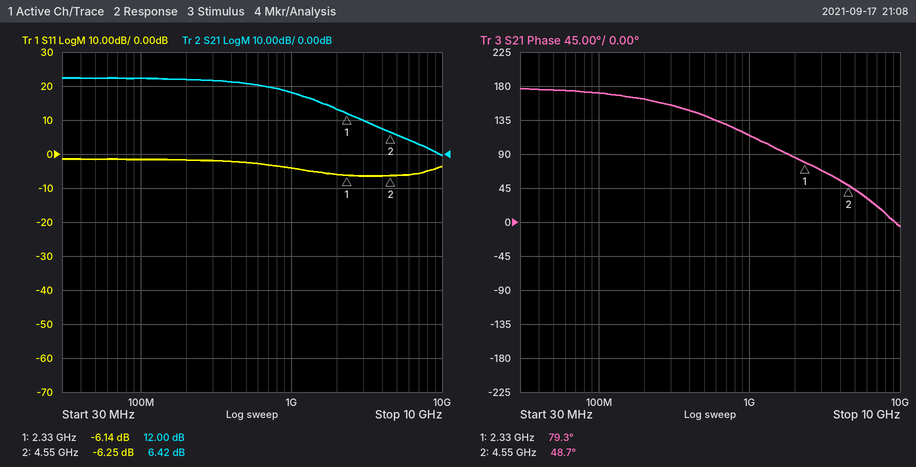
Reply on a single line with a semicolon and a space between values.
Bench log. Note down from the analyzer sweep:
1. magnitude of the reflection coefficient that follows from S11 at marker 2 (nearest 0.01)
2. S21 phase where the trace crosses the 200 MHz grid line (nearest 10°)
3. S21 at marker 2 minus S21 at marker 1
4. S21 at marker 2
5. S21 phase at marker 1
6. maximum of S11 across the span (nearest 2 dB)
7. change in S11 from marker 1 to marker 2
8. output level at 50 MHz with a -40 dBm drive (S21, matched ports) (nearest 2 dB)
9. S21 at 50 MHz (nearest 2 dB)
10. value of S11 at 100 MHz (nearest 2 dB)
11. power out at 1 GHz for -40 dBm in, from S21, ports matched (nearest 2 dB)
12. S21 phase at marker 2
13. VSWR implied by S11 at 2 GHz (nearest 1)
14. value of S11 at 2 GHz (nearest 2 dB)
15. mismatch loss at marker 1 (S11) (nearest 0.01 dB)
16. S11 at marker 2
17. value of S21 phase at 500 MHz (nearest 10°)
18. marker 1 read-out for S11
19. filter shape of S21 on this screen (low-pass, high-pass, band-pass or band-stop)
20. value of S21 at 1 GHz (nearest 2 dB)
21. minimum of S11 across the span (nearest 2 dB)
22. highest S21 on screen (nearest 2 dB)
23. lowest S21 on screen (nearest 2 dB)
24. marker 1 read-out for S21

0.49; 160°; -5.58 dB; 6.42 dB; 79.3°; -2 dB; -0.11 dB; -18 dBm; 22 dB; -2 dB; -22 dBm; 48.7°; 3; -6 dB; 1.21 dB; -6.25 dB; 140°; -6.14 dB; low-pass; 18 dB; -6 dB; 22 dB; 0 dB; 12.00 dB
